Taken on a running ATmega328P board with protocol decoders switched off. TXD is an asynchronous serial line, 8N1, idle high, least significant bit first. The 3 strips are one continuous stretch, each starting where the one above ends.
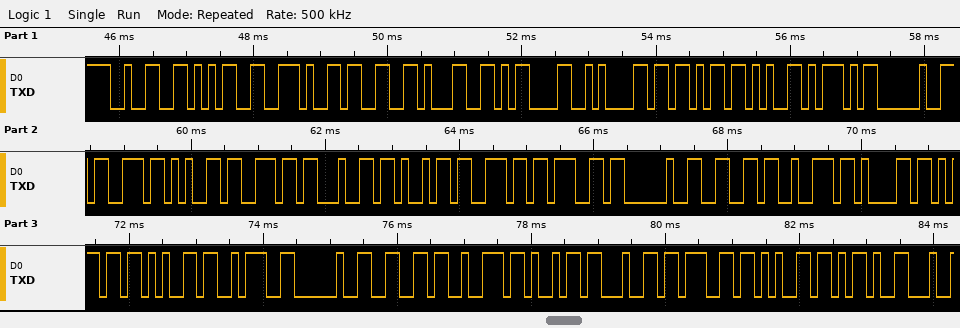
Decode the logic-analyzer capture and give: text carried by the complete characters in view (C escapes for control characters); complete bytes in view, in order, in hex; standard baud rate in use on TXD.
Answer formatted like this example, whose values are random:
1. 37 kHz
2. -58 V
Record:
1. "25.31\r\n[+] sending frame: fridge-"
2. 32 35 2E 33 31 0D 0A 5B 2B 5D 20 73 65 6E 64 69 6E 67 20 66 72 61 6D 65 3A 20 66 72 69 64 67 65 2D
3. 9600 baud
